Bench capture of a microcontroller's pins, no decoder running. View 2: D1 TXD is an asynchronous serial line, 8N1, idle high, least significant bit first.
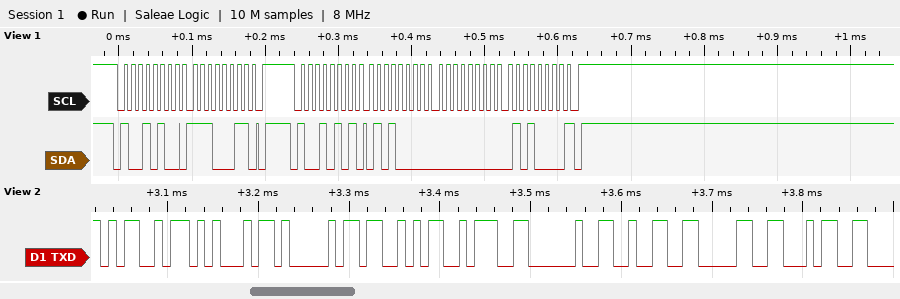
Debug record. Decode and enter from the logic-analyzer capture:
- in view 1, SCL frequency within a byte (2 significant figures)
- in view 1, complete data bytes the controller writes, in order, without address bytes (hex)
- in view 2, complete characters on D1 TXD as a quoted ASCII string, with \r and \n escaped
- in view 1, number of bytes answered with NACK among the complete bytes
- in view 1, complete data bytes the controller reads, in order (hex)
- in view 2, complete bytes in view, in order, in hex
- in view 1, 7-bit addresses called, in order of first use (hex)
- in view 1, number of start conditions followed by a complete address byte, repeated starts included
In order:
100 kHz
E3
"MEAS: 204"
1
50 00 50
4D 45 41 53 3A 20 32 30 34
0x4A
2
